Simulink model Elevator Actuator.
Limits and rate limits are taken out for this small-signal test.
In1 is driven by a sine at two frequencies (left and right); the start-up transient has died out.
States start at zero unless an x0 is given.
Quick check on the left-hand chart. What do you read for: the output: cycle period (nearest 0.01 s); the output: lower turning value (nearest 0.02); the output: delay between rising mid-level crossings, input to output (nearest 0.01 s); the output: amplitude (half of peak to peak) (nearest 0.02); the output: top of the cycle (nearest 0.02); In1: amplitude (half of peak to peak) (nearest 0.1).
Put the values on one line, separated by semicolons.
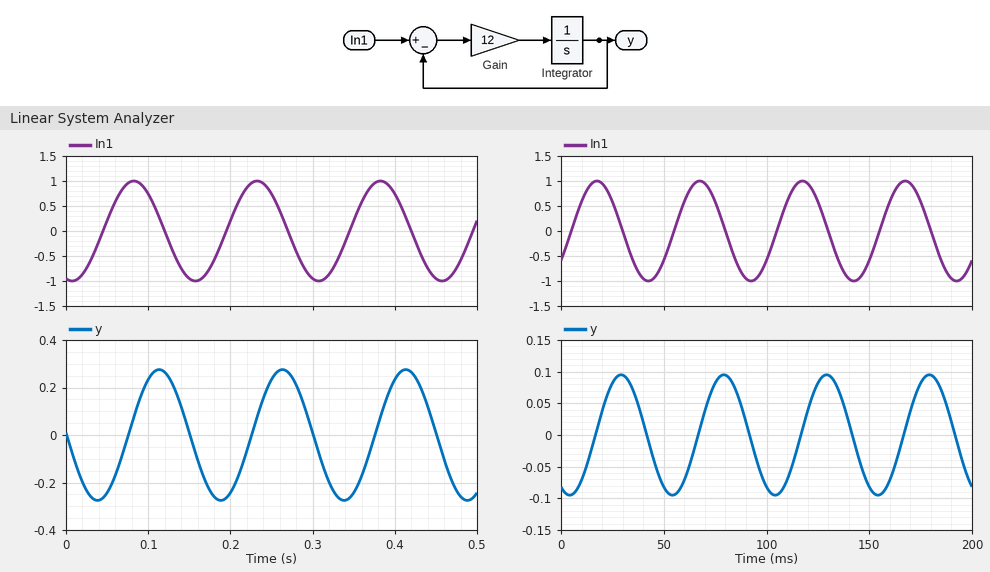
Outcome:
0.15 s; -0.28; 0.03 s; 0.28; 0.28; 1.0
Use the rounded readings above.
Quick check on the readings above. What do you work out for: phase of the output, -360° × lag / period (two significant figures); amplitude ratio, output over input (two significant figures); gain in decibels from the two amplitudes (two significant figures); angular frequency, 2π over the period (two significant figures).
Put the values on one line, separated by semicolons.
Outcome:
-72°; 0.28; -11 dB; 42 rad/s
